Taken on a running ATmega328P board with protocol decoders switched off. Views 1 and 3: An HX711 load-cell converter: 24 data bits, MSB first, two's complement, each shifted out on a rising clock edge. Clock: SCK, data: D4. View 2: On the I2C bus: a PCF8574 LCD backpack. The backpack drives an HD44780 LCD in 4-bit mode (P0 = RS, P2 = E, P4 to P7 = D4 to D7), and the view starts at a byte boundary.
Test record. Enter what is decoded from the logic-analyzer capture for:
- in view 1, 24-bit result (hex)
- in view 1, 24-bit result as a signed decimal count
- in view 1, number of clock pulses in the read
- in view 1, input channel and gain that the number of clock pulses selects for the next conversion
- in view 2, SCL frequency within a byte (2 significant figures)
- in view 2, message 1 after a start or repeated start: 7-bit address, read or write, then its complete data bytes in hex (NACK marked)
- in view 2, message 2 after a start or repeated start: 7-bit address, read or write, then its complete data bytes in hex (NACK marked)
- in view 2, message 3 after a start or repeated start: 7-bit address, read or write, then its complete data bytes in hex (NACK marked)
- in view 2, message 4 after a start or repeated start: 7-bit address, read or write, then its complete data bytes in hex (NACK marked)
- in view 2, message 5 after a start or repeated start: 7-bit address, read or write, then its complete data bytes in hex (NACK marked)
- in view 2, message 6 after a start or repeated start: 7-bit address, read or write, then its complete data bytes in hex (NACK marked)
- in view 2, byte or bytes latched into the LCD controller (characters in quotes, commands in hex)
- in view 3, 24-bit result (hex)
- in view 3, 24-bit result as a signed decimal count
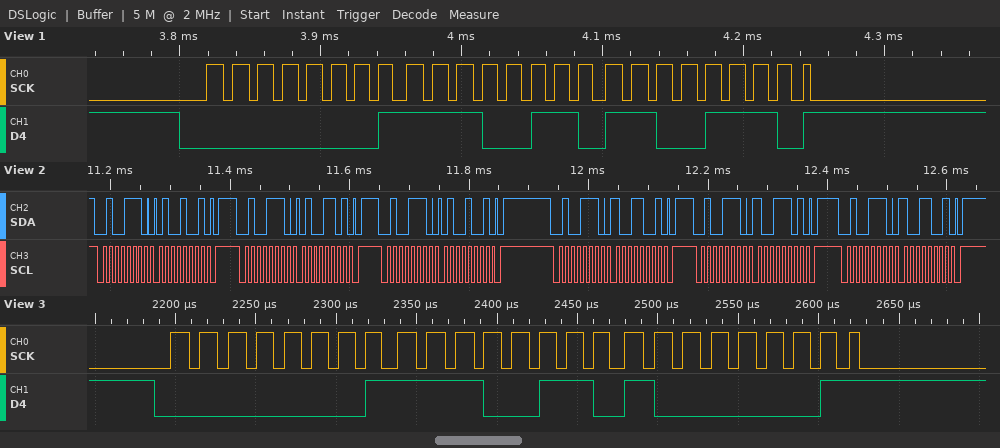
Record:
0x01E6CE
124622
25
channel A, gain 128
100 kHz
0x27 write: 49
0x27 write: 4D
0x27 write: 49
0x27 write: 99
0x27 write: 9D
0x27 write: 99
'I'
0x01E681
124545
